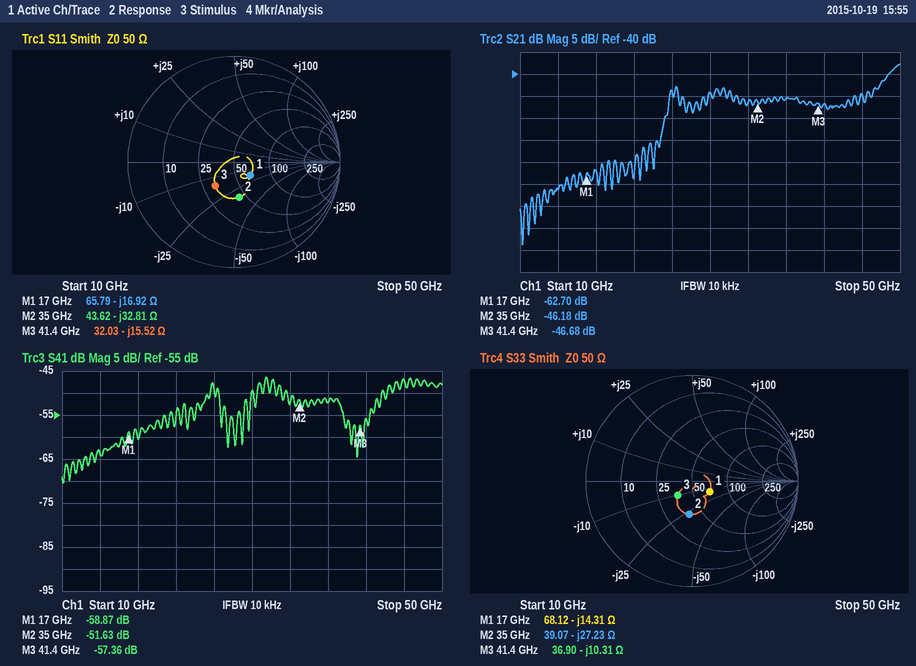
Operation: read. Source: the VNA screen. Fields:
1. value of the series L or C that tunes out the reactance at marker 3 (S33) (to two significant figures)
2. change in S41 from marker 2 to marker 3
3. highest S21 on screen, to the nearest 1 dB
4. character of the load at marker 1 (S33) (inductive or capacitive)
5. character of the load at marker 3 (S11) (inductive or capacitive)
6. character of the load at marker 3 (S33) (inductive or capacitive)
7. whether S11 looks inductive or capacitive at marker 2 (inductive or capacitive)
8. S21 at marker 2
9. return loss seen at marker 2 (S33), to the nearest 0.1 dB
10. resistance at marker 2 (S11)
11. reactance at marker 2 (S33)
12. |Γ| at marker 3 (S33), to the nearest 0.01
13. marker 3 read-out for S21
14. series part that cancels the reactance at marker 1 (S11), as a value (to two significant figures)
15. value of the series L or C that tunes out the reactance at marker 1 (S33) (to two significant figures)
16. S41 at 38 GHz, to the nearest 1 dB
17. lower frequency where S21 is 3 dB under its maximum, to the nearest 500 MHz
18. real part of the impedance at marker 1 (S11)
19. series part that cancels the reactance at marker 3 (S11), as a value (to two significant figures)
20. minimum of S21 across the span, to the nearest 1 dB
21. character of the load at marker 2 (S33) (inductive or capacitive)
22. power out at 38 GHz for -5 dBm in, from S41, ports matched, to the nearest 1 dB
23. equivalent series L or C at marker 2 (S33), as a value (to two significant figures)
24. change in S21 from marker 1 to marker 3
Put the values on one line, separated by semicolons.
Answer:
40 pH; -5.73 dB; -38 dB; capacitive; capacitive; capacitive; capacitive; -46.18 dB; 10.0 dB; 43.62 Ω; -27.23 Ω; 0.19; -46.68 dB; 160 pH; 130 pH; -52 dB; 48.5 GHz; 65.79 Ω; 60 pH; -79 dB; capacitive; -57 dBm; 170 fF; 16.02 dB
